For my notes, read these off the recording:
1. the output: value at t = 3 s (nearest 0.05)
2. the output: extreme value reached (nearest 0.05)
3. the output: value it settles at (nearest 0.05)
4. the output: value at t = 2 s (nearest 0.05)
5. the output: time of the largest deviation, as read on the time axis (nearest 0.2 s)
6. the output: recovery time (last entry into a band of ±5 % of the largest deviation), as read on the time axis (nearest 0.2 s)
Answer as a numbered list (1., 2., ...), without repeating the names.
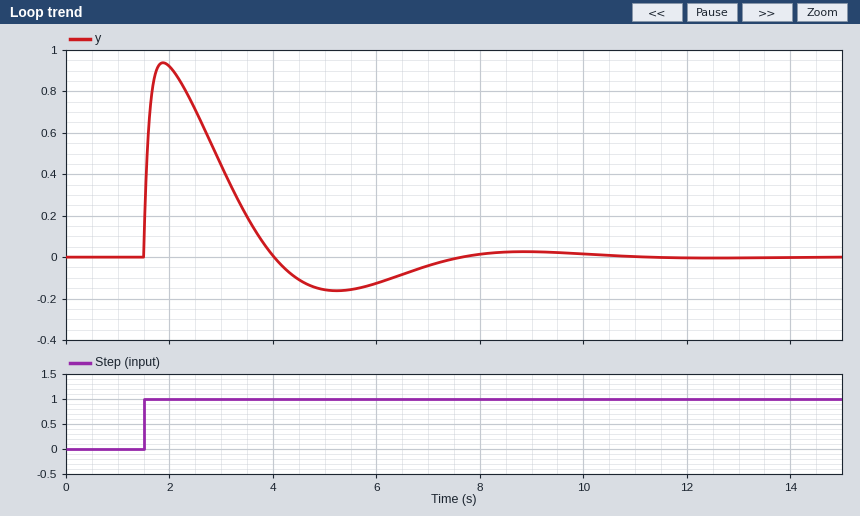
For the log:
1. 0.45
2. 0.95
3. 0.00
4. 0.90
5. 1.8 s
6. 7.0 s
